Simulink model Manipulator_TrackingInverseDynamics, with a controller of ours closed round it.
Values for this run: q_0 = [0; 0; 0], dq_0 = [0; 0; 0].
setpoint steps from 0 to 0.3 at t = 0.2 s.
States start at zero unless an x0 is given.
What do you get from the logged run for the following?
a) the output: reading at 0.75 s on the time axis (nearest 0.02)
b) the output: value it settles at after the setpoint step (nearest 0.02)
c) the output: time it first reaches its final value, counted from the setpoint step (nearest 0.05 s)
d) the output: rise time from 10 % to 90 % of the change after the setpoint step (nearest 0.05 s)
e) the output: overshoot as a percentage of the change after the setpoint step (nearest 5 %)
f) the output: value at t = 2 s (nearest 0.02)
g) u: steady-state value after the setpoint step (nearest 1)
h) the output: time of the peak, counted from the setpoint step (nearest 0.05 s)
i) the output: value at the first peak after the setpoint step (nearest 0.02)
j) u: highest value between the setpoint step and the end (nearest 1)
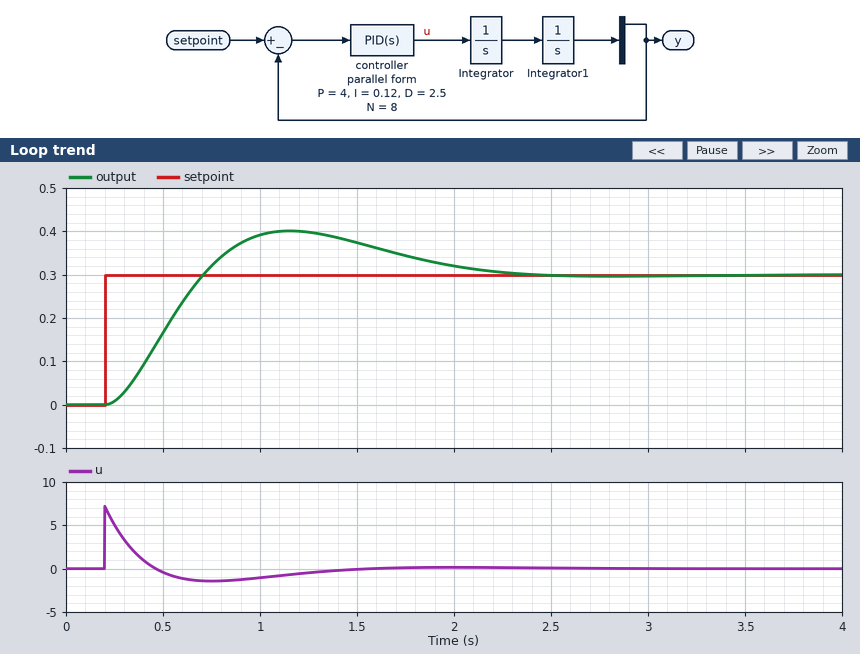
0.32
0.30
0.50 s
0.35 s
35 %
0.32
0
0.95 s
0.40
7
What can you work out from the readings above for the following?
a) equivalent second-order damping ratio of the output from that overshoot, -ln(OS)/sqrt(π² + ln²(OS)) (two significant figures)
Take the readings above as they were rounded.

0.32
